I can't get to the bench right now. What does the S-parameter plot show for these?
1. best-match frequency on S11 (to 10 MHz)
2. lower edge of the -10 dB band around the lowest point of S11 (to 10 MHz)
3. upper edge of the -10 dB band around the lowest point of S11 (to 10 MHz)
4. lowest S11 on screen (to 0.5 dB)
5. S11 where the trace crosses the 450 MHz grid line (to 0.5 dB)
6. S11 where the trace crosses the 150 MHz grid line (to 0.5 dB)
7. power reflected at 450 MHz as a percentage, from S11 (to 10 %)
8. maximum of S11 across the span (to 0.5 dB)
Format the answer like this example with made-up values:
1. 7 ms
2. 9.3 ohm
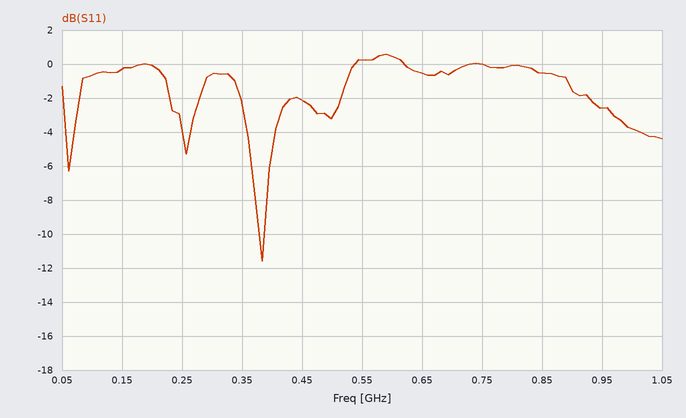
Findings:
1. 380 MHz
2. 380 MHz
3. 390 MHz
4. -11.5 dB
5. -2.0 dB
6. -0.5 dB
7. 60 %
8. 0.5 dB
